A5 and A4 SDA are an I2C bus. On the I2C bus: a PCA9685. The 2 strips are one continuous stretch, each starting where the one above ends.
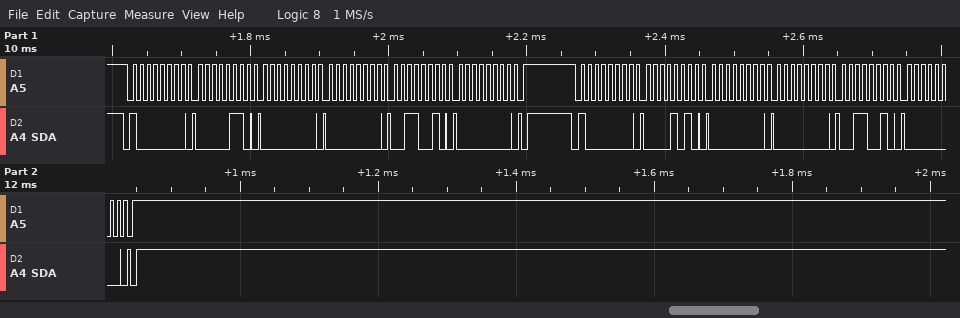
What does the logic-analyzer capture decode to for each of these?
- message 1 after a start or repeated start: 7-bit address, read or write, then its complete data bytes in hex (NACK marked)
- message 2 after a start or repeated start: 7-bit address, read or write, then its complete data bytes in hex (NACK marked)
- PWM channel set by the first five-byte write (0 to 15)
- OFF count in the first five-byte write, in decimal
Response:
0x40 write: 06 00 00 32 00
0x40 write: 0A 00 00 32 00
0
50
